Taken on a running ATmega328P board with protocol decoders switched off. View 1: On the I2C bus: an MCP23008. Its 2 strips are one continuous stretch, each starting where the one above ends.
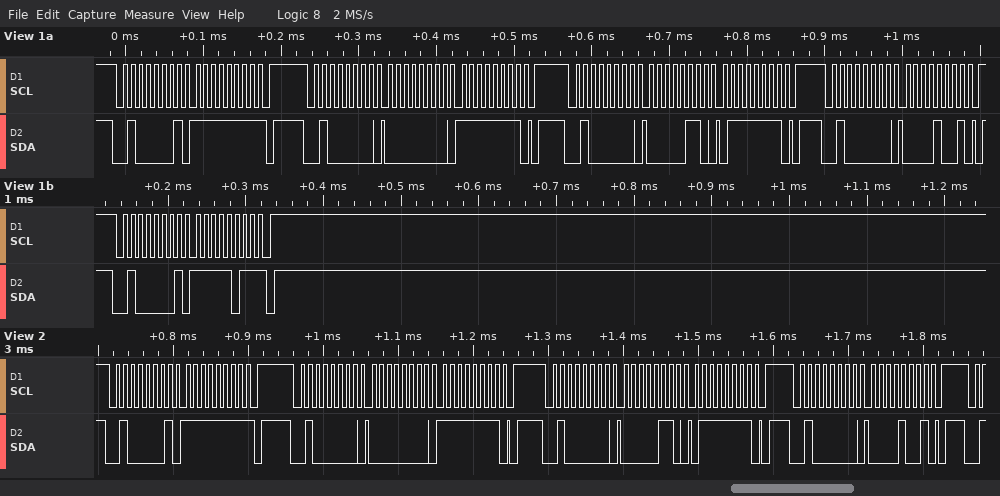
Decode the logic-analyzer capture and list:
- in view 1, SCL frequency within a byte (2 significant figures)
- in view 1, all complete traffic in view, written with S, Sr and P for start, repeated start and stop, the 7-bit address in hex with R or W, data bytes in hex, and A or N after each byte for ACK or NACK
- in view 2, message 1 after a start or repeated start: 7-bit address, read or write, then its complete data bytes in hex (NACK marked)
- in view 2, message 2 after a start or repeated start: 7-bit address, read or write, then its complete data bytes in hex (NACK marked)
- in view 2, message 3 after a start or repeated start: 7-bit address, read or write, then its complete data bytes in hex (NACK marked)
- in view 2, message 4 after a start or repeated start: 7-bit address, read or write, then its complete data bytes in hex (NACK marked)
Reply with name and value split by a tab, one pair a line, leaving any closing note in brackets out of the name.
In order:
in view 1, SCL frequency within a byte	100 kHz
in view 1, all complete traffic in view, written with S, Sr and P for start, repeated start and stop, the 7-bit address in hex with R or W, data bytes in hex, and A or N after each byte for ACK or NACK	S 20R A FF N P S 20W A 00 A FF A P S 20W A 06 A 7F A P S 20W A 09 A P S 20R A FB N P
in view 2, message 1 after a start or repeated start: 7-bit address, read or write, then its complete data bytes in hex	0x20 read: FF NACK
in view 2, message 2 after a start or repeated start: 7-bit address, read or write, then its complete data bytes in hex	0x20 write: 00 FF
in view 2, message 3 after a start or repeated start: 7-bit address, read or write, then its complete data bytes in hex	0x20 write: 06 7F
in view 2, message 4 after a start or repeated start: 7-bit address, read or write, then its complete data bytes in hex	0x20 write: 09
